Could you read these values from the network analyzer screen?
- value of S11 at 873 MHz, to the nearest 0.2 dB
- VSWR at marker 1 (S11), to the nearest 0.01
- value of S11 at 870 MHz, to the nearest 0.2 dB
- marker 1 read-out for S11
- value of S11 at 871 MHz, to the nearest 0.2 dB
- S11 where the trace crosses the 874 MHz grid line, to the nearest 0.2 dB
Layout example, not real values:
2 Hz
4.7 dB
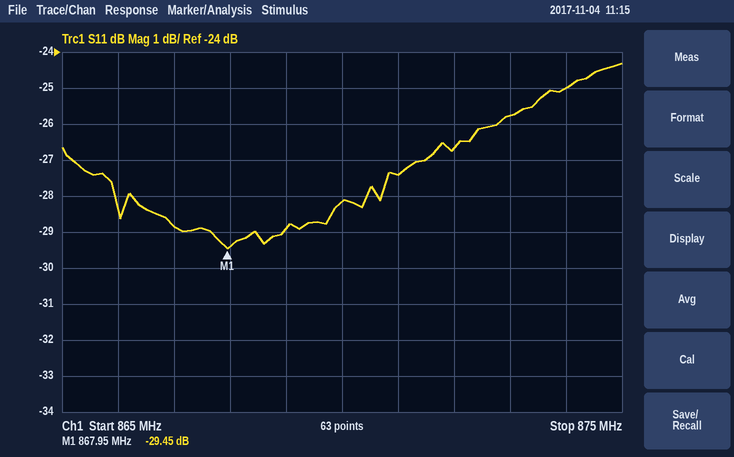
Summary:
-25.8 dB
1.07
-28.2 dB
-29.45 dB
-27.4 dB
-25.0 dB
